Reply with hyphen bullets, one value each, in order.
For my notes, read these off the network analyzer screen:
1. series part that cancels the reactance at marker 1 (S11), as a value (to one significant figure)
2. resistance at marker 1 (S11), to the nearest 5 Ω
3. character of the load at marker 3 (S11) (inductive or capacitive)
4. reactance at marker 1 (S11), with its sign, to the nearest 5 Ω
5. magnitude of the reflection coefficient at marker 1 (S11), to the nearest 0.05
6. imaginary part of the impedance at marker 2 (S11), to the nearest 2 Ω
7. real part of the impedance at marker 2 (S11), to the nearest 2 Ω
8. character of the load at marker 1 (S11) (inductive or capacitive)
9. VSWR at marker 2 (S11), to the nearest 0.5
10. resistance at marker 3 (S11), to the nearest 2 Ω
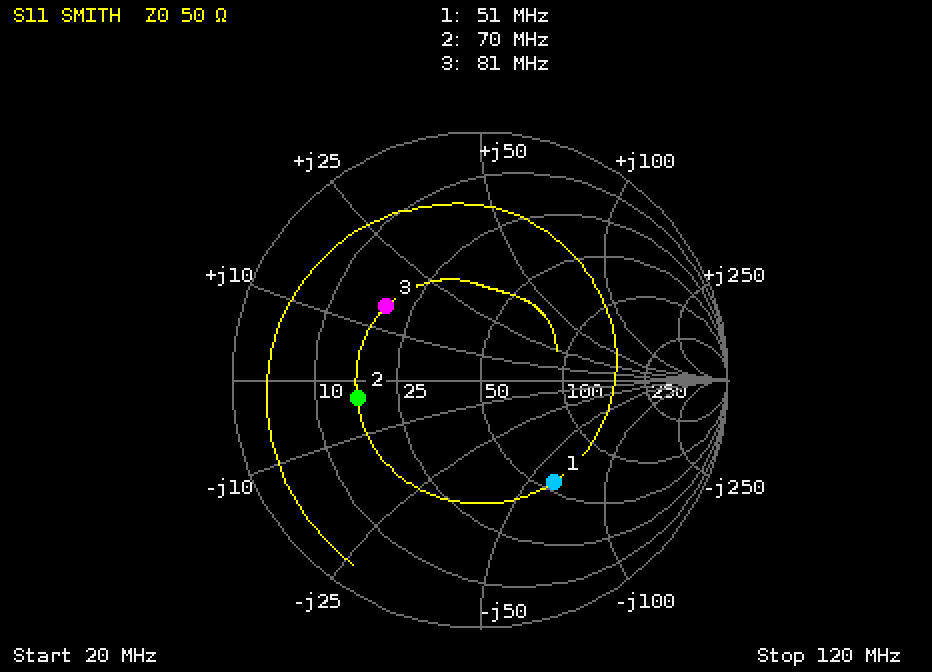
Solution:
- 200 nH
- 55 Ω
- inductive
- -60 Ω
- 0.50
- -4 Ω
- 16 Ω
- capacitive
- 3.0
- 20 Ω
